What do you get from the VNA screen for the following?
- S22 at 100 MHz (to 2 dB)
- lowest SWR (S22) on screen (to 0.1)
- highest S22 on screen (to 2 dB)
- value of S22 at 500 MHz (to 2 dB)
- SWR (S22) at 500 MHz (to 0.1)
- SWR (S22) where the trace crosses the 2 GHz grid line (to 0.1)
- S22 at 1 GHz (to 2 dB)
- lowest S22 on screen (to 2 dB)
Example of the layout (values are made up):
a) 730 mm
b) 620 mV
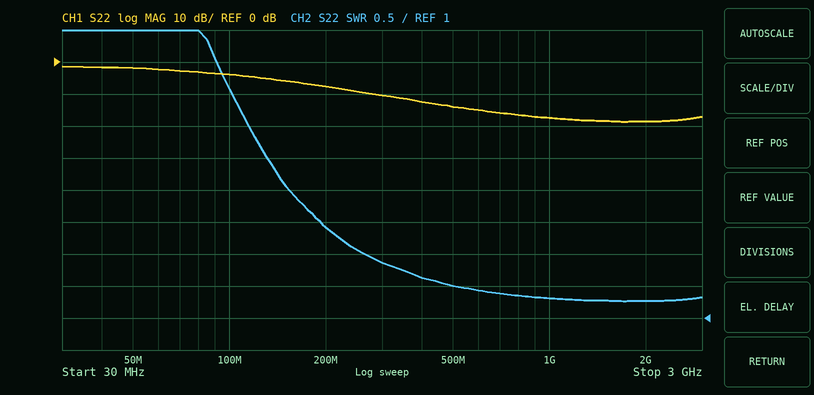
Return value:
a) -4 dB
b) 1.3
c) -2 dB
d) -14 dB
e) 1.5
f) 1.3
g) -18 dB
h) -18 dB
